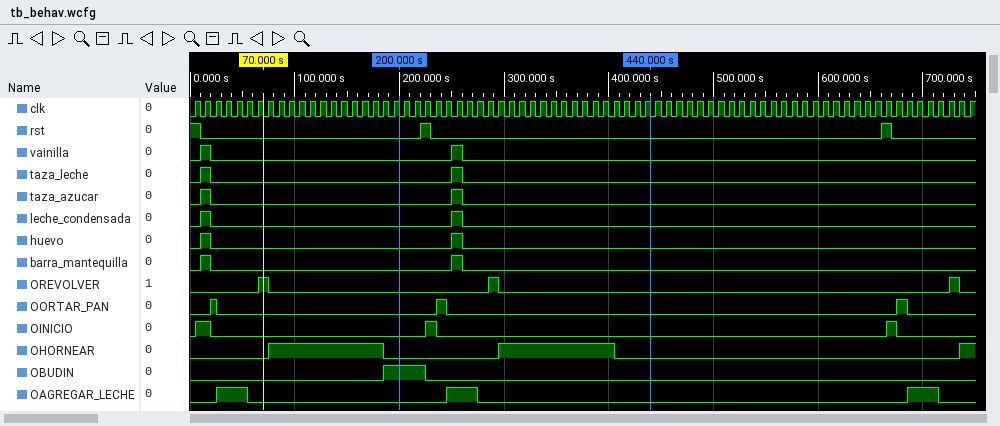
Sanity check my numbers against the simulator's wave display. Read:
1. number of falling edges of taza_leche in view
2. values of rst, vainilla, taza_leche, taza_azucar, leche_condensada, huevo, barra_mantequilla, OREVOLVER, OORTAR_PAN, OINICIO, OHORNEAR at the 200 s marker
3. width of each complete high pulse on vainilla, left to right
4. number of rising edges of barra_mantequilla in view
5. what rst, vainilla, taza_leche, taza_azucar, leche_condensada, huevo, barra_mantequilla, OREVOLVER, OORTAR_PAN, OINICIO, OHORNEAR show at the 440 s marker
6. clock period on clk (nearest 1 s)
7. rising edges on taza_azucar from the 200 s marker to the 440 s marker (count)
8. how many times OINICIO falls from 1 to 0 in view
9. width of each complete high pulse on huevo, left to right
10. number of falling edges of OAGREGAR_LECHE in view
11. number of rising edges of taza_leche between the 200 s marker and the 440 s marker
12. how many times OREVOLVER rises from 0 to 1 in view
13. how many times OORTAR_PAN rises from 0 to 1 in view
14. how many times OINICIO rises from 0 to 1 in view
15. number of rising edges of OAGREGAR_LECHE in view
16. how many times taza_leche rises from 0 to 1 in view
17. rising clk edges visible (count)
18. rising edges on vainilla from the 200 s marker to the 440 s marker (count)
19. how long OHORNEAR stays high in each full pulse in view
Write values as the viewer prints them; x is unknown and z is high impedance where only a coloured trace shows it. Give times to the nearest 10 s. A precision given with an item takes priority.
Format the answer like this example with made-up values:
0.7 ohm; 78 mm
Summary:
2; rst=0, vainilla=0, taza_leche=0, taza_azucar=0, leche_condensada=0, huevo=0, barra_mantequilla=0, OREVOLVER=0, OORTAR_PAN=0, OINICIO=0, OHORNEAR=0; 10 s, 10 s; 2; rst=0, vainilla=0, taza_leche=0, taza_azucar=0, leche_condensada=0, huevo=0, barra_mantequilla=0, OREVOLVER=0, OORTAR_PAN=0, OINICIO=0, OHORNEAR=0; 10 s; 1; 3; 10 s, 10 s; 3; 1; 3; 3; 3; 3; 2; 75; 1; 110 s, 110 s
